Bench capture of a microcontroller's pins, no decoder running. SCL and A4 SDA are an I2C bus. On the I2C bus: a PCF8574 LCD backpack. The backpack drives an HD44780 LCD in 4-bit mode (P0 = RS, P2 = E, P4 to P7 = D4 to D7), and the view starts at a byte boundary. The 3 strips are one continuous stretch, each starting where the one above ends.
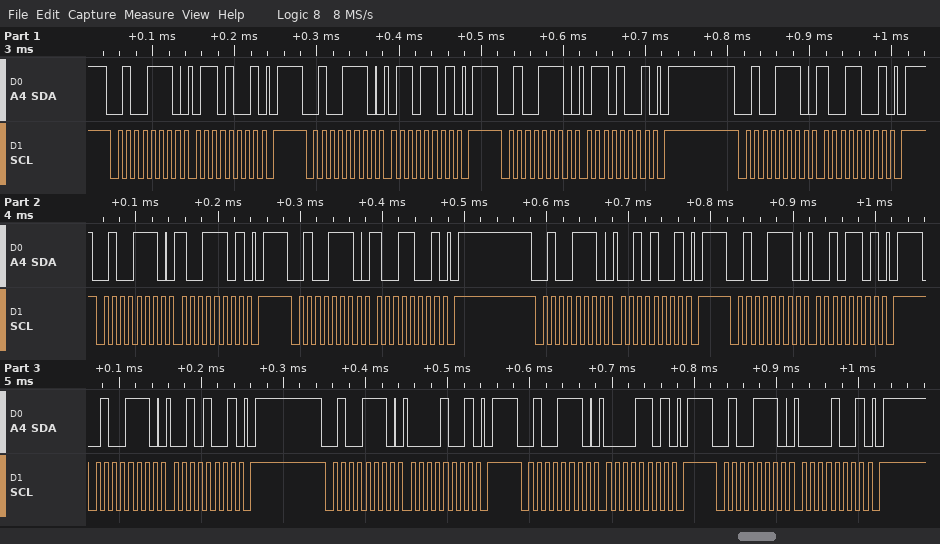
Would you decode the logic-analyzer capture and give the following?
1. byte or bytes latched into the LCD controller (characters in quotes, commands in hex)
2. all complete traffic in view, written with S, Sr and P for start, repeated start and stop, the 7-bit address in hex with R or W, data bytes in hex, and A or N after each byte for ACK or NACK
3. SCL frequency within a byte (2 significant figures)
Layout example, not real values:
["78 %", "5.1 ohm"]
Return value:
["'i' ' '", "S 27W A 69 A P S 27W A 6D A P S 27W A 69 A P S 27W A 99 A P S 27W A 9D A P S 27W A 99 A P S 27W A 29 A P S 27W A 2D A P S 27W A 29 A P S 27W A 09 A P S 27W A 0D A P S 27W A 09 A P", "100 kHz"]
